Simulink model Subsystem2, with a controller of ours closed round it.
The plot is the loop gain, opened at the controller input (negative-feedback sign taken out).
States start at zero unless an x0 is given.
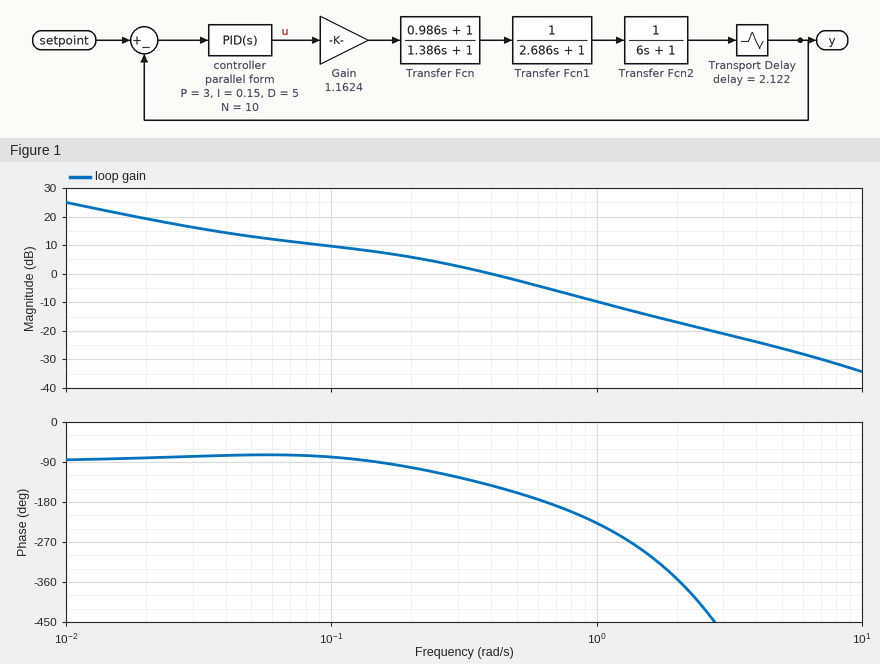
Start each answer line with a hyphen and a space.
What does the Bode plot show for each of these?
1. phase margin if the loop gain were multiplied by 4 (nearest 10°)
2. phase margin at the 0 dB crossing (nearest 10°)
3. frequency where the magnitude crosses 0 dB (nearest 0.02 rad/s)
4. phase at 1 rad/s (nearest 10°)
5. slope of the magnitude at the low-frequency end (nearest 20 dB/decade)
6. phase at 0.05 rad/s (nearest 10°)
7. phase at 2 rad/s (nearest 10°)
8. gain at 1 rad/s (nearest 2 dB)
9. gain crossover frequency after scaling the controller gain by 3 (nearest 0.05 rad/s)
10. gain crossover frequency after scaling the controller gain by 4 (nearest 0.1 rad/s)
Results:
- -80°
- 40°
- 0.40 rad/s
- -230°
- -20 dB/decade
- -70°
- -350°
- -10 dB
- 1.00 rad/s
- 1.2 rad/s
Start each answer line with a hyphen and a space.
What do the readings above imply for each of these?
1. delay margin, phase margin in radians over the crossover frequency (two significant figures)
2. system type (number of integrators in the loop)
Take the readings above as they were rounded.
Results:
- 1.7 s
- 1
